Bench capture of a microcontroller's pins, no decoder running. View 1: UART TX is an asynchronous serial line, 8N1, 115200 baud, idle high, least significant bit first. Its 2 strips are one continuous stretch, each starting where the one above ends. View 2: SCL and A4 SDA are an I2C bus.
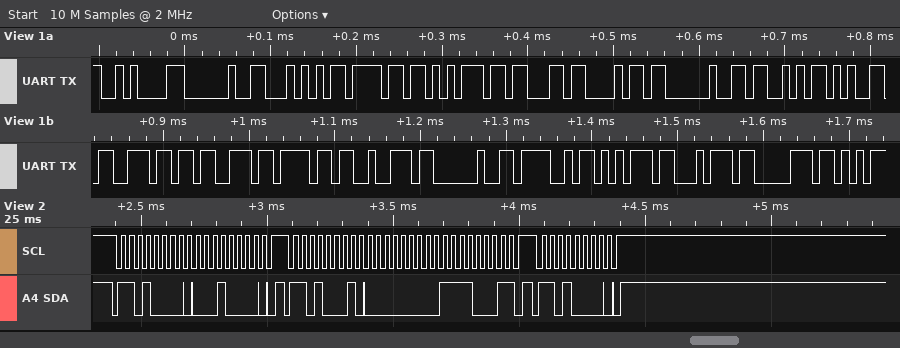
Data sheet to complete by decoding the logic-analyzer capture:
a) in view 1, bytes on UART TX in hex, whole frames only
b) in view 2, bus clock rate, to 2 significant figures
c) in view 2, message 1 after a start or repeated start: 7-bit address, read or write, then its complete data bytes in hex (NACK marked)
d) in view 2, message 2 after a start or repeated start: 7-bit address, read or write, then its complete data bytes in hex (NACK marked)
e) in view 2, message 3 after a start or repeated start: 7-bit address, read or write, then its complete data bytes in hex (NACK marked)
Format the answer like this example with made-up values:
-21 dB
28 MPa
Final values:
0A 20 54 6F 75 63 68 20 53 65 6E 73 6F 72 20 4F 75 74 70
31 kHz
0x68 write: 10
0x68 read: 00 F1 NACK
0x68 write
